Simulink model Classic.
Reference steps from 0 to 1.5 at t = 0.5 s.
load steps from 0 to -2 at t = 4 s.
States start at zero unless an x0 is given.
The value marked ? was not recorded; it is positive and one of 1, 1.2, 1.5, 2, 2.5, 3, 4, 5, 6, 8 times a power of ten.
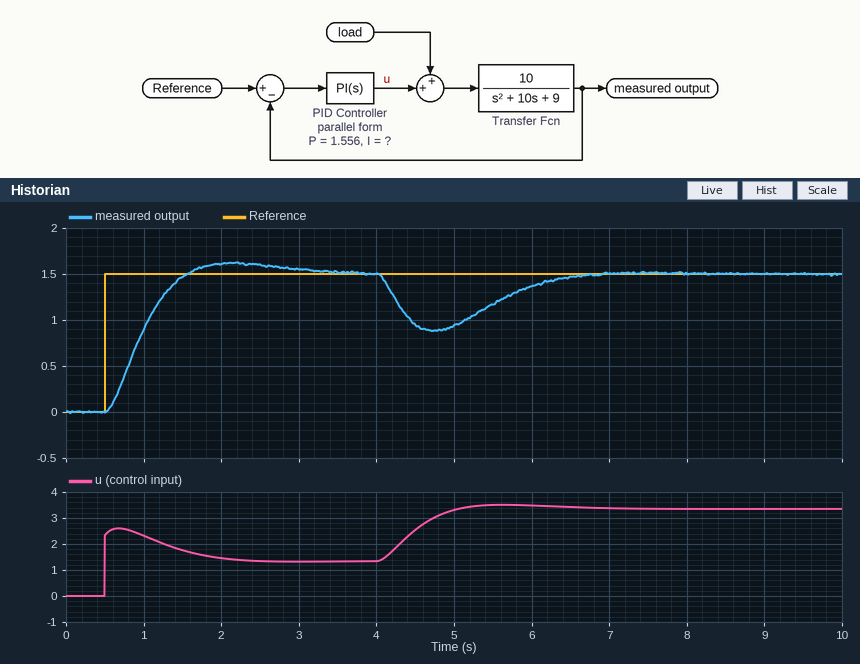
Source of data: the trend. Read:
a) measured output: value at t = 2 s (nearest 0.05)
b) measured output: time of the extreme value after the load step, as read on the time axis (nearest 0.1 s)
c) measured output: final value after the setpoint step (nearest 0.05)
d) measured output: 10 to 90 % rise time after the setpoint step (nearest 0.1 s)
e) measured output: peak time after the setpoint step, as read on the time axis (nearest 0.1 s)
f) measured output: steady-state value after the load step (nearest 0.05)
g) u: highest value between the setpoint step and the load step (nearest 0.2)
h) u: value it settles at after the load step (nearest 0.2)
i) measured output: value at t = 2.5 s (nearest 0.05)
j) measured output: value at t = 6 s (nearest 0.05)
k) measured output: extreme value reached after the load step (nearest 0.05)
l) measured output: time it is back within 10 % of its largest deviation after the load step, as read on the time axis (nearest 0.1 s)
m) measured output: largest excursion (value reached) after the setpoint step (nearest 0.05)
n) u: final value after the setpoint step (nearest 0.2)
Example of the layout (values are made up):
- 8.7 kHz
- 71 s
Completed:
- 1.60
- 4.7 s
- 1.50
- 0.7 s
- 2.1 s
- 1.50
- 2.6
- 3.4
- 1.60
- 1.35
- 0.90
- 6.3 s
- 1.60
- 1.4
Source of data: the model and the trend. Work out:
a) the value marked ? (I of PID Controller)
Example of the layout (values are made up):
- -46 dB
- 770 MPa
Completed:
- 2.5
